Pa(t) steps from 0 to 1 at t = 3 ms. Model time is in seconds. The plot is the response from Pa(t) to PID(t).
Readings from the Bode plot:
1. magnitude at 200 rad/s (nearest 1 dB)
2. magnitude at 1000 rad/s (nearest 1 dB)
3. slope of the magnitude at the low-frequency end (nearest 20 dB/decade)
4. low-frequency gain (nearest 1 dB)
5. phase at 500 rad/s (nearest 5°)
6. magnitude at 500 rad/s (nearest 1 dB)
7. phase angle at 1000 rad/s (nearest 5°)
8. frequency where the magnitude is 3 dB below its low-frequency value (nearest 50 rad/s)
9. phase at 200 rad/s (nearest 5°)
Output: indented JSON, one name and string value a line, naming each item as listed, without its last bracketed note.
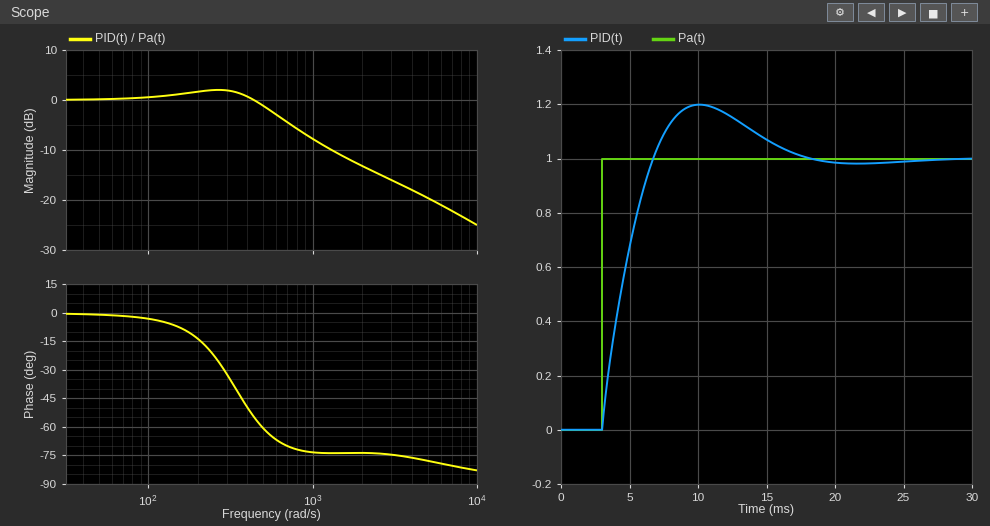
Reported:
{
  "magnitude at 200 rad/s": "2 dB",
  "magnitude at 1000 rad/s": "-8 dB",
  "slope of the magnitude at the low-frequency end": "0 dB/decade",
  "low-frequency gain": "0 dB",
  "phase at 500 rad/s": "-60°",
  "magnitude at 500 rad/s": "-1 dB",
  "phase angle at 1000 rad/s": "-75°",
  "frequency where the magnitude is 3 dB below its low-frequency value": "600 rad/s",
  "phase at 200 rad/s": "-15°"
}
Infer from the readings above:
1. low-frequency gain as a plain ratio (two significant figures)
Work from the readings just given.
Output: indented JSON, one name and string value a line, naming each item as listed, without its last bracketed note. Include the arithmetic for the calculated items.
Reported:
{
  "low-frequency gain as a plain ratio": "10^(0 / 20) = 1.0"
}
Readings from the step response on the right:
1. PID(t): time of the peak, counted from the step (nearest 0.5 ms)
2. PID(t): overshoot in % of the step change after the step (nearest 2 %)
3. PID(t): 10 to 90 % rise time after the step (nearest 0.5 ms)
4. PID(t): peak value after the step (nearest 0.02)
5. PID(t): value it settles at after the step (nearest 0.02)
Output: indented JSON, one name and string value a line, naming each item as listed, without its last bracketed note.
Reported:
{
  "PID(t): time of the peak, counted from the step": "7.0 ms",
  "PID(t): overshoot in % of the step change after the step": "20 %",
  "PID(t): 10 to 90 % rise time after the step": "3.0 ms",
  "PID(t): peak value after the step": "1.20",
  "PID(t): value it settles at after the step": "1.00"
}
